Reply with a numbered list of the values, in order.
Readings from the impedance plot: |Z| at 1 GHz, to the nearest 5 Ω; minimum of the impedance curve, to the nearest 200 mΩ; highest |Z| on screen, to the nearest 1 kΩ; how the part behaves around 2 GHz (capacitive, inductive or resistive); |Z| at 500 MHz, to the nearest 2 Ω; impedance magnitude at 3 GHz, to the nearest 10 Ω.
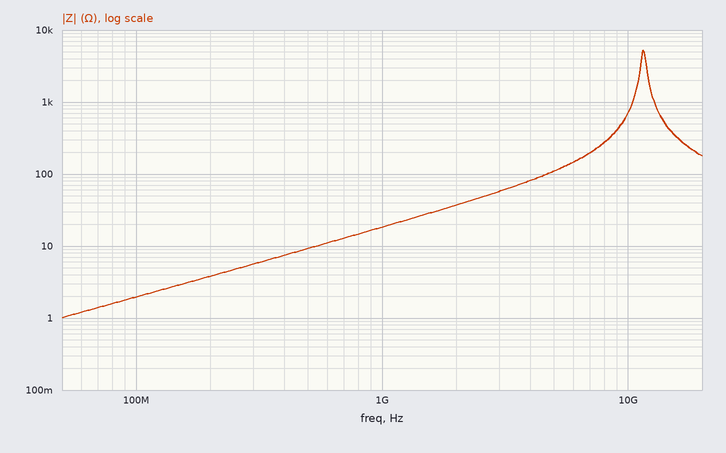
1. 20 Ω
2. 1.0 Ω
3. 5 kΩ
4. inductive
5. 10 Ω
6. 60 Ω
